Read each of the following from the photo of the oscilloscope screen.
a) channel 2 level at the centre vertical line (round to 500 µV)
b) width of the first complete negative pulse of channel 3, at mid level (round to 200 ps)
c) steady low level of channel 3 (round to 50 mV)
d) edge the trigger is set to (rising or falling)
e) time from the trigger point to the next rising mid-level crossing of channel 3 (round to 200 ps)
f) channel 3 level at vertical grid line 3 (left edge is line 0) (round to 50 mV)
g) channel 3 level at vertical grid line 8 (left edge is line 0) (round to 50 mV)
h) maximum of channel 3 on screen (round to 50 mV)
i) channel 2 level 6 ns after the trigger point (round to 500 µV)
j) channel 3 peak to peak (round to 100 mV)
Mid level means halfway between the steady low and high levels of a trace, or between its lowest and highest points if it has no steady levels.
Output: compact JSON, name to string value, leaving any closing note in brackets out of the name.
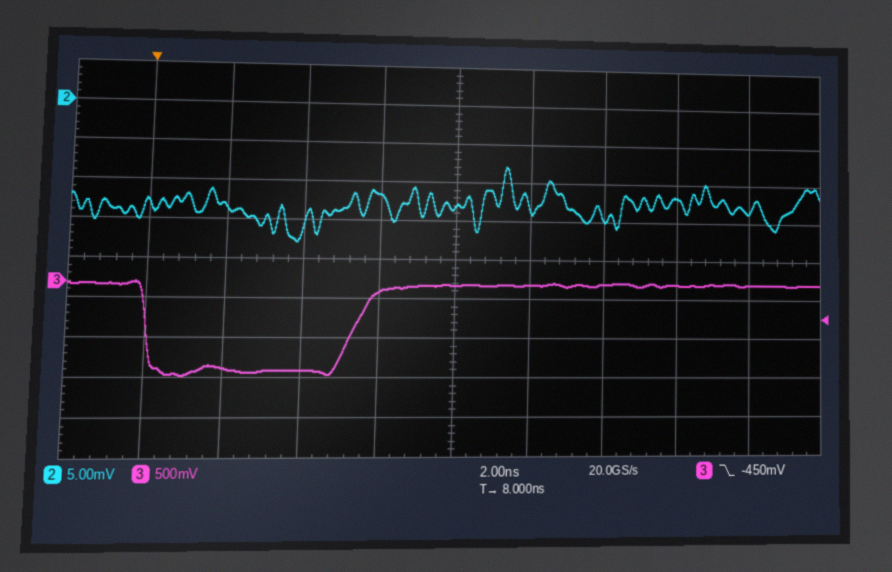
{"channel 2 level at the centre vertical line": "-13.0 mV", "width of the first complete negative pulse of channel 3, at mid level": "5.4 ns", "steady low level of channel 3": "-1.10 V", "edge the trigger is set to": "falling", "time from the trigger point to the next rising mid-level crossing of channel 3": "5.4 ns", "channel 3 level at vertical grid line 3 (left edge is line 0)": "-1.10 V", "channel 3 level at vertical grid line 8 (left edge is line 0)": "0 mV", "maximum of channel 3 on screen": "0 mV", "channel 2 level 6 ns after the trigger point": "-12.0 mV", "channel 3 peak to peak": "1.20 V"}
